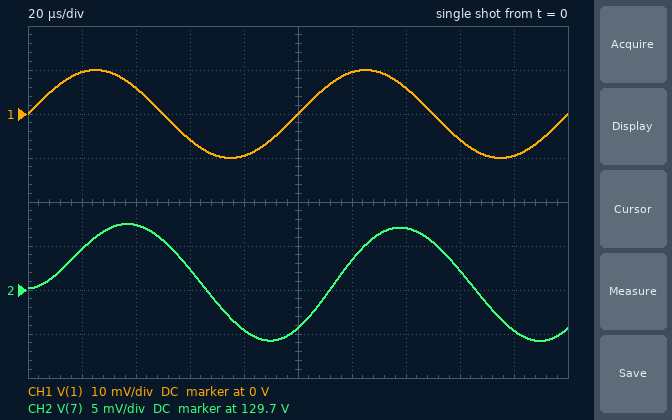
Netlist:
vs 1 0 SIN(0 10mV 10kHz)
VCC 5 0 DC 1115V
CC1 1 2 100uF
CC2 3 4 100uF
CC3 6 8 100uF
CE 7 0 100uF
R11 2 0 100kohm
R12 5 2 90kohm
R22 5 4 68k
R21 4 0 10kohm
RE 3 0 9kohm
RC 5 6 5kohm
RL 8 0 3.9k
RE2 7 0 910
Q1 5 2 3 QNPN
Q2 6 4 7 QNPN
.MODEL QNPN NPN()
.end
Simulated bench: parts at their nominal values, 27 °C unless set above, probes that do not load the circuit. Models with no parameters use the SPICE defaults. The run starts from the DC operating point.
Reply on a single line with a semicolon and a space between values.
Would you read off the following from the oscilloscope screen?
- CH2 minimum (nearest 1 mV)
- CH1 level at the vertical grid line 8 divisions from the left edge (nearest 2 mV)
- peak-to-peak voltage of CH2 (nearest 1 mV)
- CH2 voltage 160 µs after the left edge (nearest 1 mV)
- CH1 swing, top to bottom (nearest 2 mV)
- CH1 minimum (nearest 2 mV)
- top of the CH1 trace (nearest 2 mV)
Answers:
129.734 V; -6 mV; 13 mV; 129.742 V; 20 mV; -10 mV; 10 mV
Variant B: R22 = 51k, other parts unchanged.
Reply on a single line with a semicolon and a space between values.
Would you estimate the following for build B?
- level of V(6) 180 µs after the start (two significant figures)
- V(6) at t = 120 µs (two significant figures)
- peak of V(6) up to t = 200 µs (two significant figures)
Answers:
250 V; 170 V; 300 V
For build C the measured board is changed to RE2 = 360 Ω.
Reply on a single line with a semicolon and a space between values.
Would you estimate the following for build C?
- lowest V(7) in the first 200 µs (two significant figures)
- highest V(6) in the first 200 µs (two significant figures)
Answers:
77 V; 140 V
